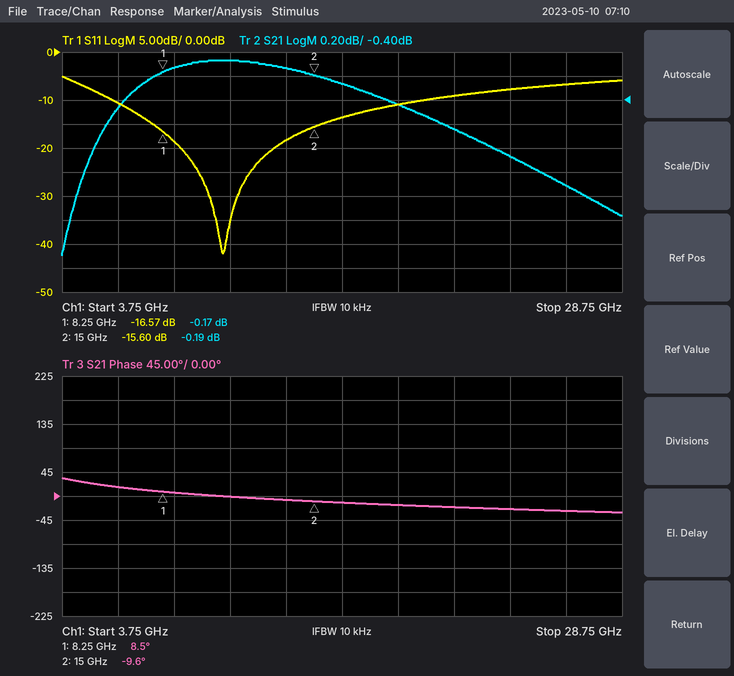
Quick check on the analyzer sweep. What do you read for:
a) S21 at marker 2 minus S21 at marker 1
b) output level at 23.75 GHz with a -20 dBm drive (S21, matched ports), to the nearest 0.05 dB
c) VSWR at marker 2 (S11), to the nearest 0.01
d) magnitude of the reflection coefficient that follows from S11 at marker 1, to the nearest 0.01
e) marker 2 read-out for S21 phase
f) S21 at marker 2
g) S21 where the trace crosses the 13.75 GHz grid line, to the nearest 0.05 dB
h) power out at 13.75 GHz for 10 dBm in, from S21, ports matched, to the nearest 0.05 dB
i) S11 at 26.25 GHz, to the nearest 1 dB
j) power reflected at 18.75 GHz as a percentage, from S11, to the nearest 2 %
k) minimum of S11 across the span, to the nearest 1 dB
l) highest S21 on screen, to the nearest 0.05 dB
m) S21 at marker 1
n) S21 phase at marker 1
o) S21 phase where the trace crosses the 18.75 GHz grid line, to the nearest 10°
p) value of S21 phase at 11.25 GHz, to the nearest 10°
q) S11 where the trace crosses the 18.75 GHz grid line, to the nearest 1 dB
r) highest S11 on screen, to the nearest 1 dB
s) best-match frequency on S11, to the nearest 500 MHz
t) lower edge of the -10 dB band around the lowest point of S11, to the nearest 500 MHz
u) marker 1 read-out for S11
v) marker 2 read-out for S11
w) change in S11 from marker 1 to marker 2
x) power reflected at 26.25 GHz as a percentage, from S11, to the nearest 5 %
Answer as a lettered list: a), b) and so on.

a) -0.02 dB
b) -20.85 dBm
c) 1.40
d) 0.15
e) -9.6°
f) -0.19 dB
g) -0.15 dB
h) 9.85 dBm
i) -7 dB
j) 8 %
k) -42 dB
l) -0.05 dB
m) -0.17 dB
n) 8.5°
o) -20°
p) 0°
q) -11 dB
r) -5 dB
s) 11.0 GHz
t) 6.0 GHz
u) -16.57 dB
v) -15.60 dB
w) 0.97 dB
x) 20 %
